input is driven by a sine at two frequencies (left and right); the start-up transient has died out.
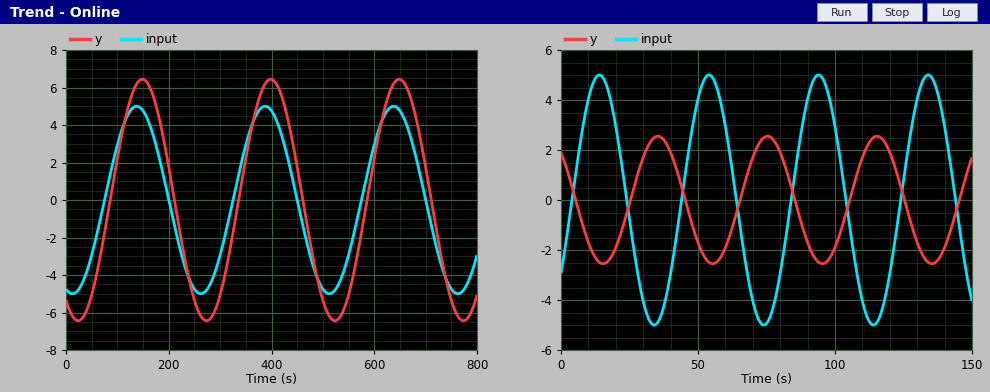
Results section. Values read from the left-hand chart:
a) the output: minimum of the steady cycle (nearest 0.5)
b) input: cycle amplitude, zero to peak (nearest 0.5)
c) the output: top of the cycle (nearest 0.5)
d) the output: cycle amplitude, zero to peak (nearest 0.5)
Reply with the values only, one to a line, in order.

-6.5
5.0
6.5
6.5
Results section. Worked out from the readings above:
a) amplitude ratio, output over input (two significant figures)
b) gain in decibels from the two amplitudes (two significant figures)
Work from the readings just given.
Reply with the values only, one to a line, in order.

1.3
2.3 dB
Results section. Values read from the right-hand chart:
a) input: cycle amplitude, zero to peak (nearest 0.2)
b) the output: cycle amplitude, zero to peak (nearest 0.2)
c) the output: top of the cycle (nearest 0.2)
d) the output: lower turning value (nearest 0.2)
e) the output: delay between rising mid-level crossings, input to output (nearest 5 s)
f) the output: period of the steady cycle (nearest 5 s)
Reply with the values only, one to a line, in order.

5.0
2.6
2.6
-2.6
20 s
40 s
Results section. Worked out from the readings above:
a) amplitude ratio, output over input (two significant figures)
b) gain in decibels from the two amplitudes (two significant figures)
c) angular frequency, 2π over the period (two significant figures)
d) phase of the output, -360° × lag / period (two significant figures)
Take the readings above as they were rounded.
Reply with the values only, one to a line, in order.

0.52
-5.7 dB
0.16 rad/s
-180°
